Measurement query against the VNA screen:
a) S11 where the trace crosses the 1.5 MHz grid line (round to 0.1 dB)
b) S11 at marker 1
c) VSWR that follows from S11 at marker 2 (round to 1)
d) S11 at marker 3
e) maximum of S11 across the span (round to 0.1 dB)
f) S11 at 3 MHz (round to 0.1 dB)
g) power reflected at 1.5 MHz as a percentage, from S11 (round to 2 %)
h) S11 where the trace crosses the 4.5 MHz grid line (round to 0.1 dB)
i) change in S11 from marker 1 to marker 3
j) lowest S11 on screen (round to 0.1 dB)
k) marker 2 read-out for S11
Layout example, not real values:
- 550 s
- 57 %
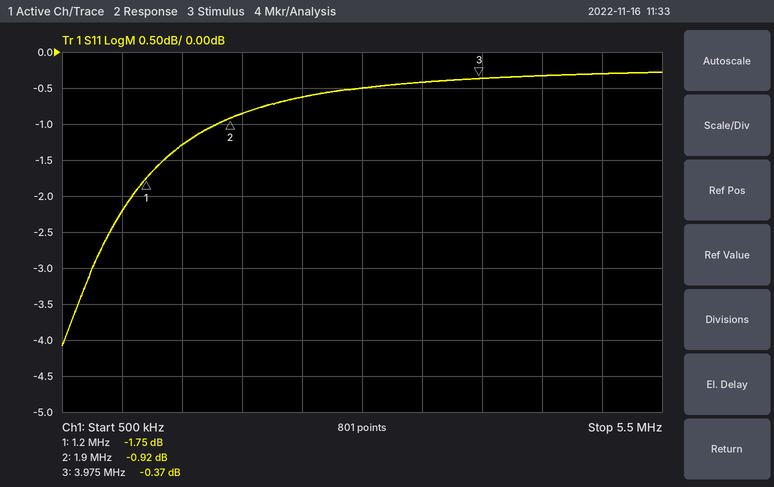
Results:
- -1.3 dB
- -1.75 dB
- 19
- -0.37 dB
- -0.3 dB
- -0.5 dB
- 74 %
- -0.3 dB
- 1.38 dB
- -4.1 dB
- -0.92 dB
